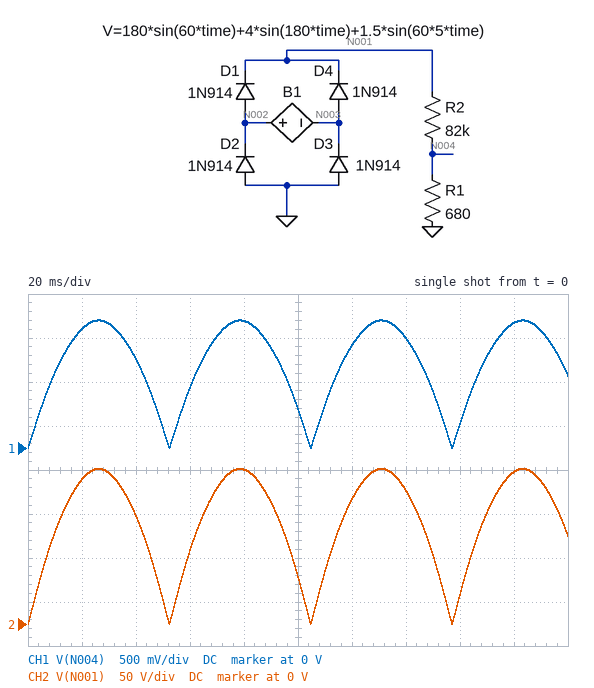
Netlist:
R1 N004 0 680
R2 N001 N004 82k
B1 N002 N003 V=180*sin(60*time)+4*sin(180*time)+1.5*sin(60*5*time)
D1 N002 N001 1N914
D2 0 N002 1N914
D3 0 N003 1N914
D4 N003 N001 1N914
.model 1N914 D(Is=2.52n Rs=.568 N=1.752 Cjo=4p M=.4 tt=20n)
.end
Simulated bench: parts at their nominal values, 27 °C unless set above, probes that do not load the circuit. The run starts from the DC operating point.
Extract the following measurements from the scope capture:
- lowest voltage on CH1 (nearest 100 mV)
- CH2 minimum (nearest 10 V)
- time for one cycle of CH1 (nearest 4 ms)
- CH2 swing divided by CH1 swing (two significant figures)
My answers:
0 V
0 V
52 ms
120
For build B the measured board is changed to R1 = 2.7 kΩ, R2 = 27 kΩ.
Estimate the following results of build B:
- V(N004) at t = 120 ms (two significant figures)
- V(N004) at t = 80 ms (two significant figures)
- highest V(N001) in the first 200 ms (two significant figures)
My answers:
13 V
16 V
180 V
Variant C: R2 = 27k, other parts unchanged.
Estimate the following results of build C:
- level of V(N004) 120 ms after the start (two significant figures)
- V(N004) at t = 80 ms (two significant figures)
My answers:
3.5 V
4.3 V
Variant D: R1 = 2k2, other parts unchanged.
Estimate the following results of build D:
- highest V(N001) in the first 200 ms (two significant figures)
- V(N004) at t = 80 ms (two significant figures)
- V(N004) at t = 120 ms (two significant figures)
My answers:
180 V
4.6 V
3.7 V
